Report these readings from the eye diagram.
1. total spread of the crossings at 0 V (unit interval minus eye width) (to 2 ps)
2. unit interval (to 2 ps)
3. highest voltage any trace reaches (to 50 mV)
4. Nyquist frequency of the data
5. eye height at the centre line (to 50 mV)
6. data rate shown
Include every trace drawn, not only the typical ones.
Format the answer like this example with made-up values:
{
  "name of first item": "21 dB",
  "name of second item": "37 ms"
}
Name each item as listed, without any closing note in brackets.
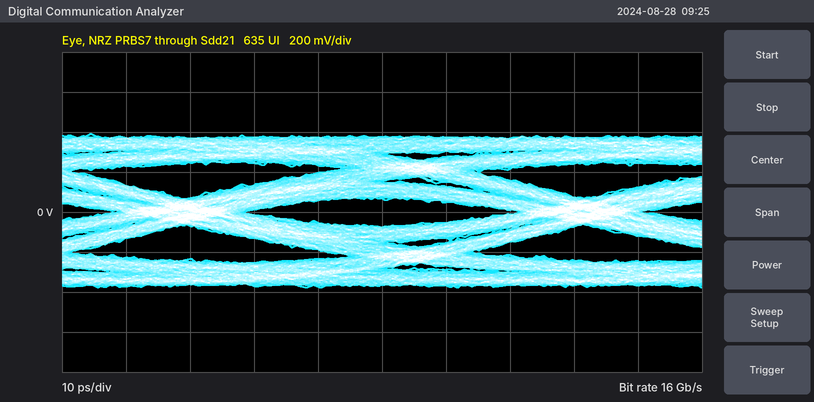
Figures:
{
  "total spread of the crossings at 0 V (unit interval minus eye width)": "20 ps",
  "unit interval": "62 ps",
  "highest voltage any trace reaches": "400 mV",
  "Nyquist frequency of the data": "8 GHz",
  "eye height at the centre line": "150 mV",
  "data rate shown": "16 Gb/s"
}
